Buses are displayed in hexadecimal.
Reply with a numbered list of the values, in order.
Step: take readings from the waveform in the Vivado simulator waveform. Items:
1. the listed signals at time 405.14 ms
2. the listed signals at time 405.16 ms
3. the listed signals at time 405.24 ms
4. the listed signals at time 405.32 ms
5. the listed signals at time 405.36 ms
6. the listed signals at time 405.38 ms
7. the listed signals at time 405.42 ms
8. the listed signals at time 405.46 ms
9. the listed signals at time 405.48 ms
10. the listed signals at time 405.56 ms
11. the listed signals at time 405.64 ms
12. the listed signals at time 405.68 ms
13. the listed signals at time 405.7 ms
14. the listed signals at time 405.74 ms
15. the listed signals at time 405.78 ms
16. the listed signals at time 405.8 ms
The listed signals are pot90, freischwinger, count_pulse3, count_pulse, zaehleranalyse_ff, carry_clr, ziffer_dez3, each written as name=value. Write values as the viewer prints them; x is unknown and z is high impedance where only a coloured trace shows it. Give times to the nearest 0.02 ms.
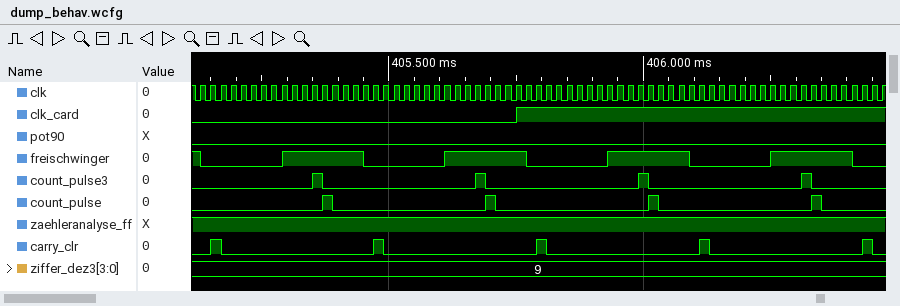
1. pot90=0, freischwinger=0, count_pulse3=0, count_pulse=0, zaehleranalyse_ff=1, carry_clr=0, ziffer_dez3=9
2. pot90=0, freischwinger=0, count_pulse3=0, count_pulse=0, zaehleranalyse_ff=1, carry_clr=1, ziffer_dez3=9
3. pot90=0, freischwinger=0, count_pulse3=0, count_pulse=0, zaehleranalyse_ff=1, carry_clr=0, ziffer_dez3=9
4. pot90=0, freischwinger=1, count_pulse3=0, count_pulse=0, zaehleranalyse_ff=1, carry_clr=0, ziffer_dez3=9
5. pot90=0, freischwinger=1, count_pulse3=1, count_pulse=0, zaehleranalyse_ff=1, carry_clr=0, ziffer_dez3=9
6. pot90=0, freischwinger=1, count_pulse3=0, count_pulse=1, zaehleranalyse_ff=1, carry_clr=0, ziffer_dez3=9
7. pot90=0, freischwinger=1, count_pulse3=0, count_pulse=0, zaehleranalyse_ff=1, carry_clr=0, ziffer_dez3=9
8. pot90=0, freischwinger=0, count_pulse3=0, count_pulse=0, zaehleranalyse_ff=1, carry_clr=0, ziffer_dez3=9
9. pot90=0, freischwinger=0, count_pulse3=0, count_pulse=0, zaehleranalyse_ff=1, carry_clr=1, ziffer_dez3=9
10. pot90=0, freischwinger=0, count_pulse3=0, count_pulse=0, zaehleranalyse_ff=1, carry_clr=0, ziffer_dez3=9
11. pot90=0, freischwinger=1, count_pulse3=0, count_pulse=0, zaehleranalyse_ff=1, carry_clr=0, ziffer_dez3=9
12. pot90=0, freischwinger=1, count_pulse3=1, count_pulse=0, zaehleranalyse_ff=1, carry_clr=0, ziffer_dez3=9
13. pot90=0, freischwinger=1, count_pulse3=0, count_pulse=1, zaehleranalyse_ff=1, carry_clr=0, ziffer_dez3=9
14. pot90=0, freischwinger=1, count_pulse3=0, count_pulse=0, zaehleranalyse_ff=1, carry_clr=0, ziffer_dez3=9
15. pot90=0, freischwinger=0, count_pulse3=0, count_pulse=0, zaehleranalyse_ff=1, carry_clr=0, ziffer_dez3=9
16. pot90=0, freischwinger=0, count_pulse3=0, count_pulse=0, zaehleranalyse_ff=1, carry_clr=1, ziffer_dez3=9
